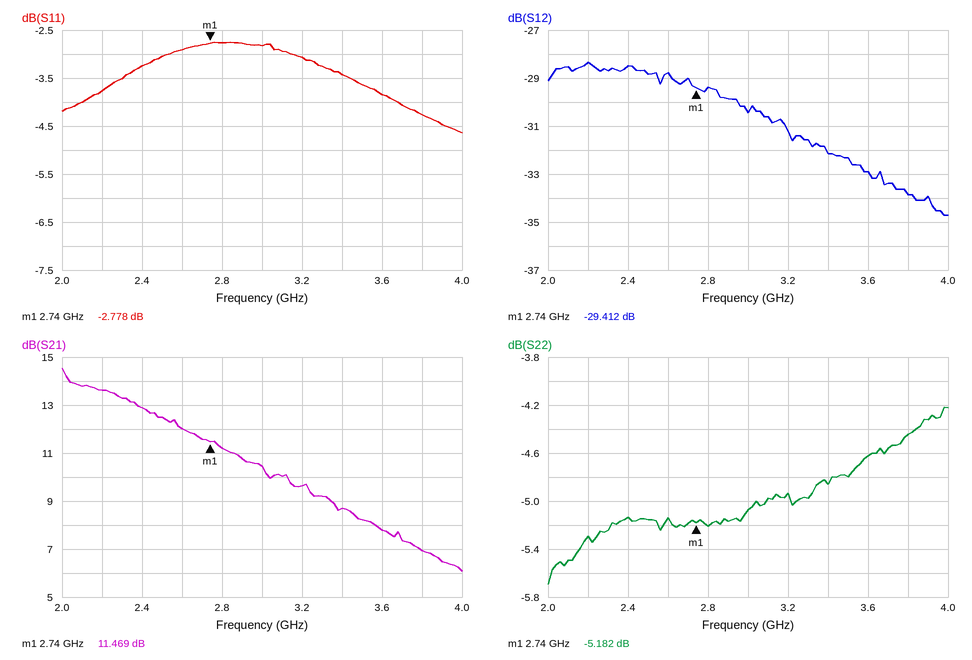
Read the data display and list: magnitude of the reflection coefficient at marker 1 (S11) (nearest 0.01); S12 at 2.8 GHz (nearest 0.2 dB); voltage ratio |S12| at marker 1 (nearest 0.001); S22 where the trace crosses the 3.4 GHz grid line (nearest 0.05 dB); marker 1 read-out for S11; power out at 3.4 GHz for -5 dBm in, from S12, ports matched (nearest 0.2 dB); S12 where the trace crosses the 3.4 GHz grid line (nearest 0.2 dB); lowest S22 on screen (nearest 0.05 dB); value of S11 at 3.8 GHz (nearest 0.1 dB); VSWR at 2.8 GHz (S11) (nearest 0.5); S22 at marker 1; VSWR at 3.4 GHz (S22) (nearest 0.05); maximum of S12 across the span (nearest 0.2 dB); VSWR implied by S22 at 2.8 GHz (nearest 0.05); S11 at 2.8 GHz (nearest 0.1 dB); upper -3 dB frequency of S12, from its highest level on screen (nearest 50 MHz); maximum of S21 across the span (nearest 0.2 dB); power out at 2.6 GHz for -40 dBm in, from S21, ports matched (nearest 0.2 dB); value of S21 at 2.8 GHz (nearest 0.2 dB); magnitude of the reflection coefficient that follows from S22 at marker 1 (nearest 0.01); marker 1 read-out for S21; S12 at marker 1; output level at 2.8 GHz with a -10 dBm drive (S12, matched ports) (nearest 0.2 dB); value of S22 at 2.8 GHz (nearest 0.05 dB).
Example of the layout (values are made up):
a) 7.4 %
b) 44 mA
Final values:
a) 0.73
b) -29.4 dB
c) 0.034
d) -4.85 dB
e) -2.778 dB
f) -37.2 dBm
g) -32.2 dB
h) -5.70 dB
i) -4.3 dB
j) 6.5
k) -5.182 dB
l) 3.65
m) -28.4 dB
n) 3.45
o) -2.8 dB
p) 3.20 GHz
q) 14.6 dB
r) -28.0 dBm
s) 11.2 dB
t) 0.55
u) 11.469 dB
v) -29.412 dB
w) -39.4 dBm
x) -5.20 dB
